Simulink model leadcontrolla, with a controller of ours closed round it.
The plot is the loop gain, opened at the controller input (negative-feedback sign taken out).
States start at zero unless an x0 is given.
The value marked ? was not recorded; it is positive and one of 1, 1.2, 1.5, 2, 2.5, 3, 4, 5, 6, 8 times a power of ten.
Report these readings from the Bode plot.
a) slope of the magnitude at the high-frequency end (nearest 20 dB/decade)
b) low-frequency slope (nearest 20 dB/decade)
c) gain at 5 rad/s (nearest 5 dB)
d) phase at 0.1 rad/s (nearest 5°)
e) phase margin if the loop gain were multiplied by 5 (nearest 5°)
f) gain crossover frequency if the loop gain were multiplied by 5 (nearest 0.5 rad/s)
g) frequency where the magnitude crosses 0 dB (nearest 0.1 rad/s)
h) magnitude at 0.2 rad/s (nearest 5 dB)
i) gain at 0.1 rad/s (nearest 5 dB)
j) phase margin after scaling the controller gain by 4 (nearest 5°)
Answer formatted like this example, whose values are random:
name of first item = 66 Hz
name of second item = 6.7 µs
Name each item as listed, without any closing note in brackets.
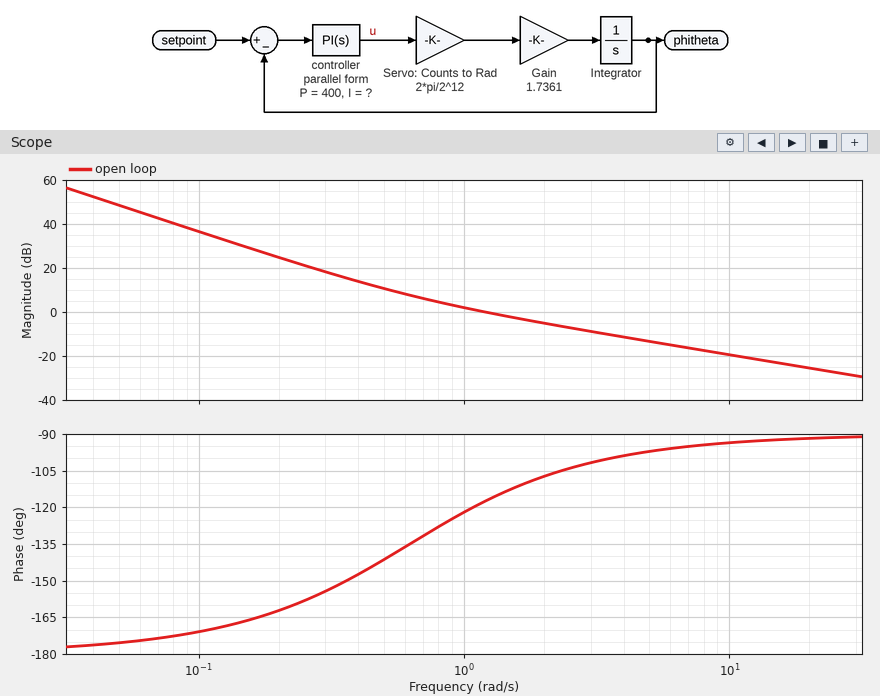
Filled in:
slope of the magnitude at the high-frequency end = -20 dB/decade
low-frequency slope = -40 dB/decade
gain at 5 rad/s = -15 dB
phase at 0.1 rad/s = -170°
phase margin if the loop gain were multiplied by 5 = 85°
gain crossover frequency if the loop gain were multiplied by 5 = 5.5 rad/s
frequency where the magnitude crosses 0 dB = 1.2 rad/s
magnitude at 0.2 rad/s = 25 dB
gain at 0.1 rad/s = 35 dB
phase margin after scaling the controller gain by 4 = 80°
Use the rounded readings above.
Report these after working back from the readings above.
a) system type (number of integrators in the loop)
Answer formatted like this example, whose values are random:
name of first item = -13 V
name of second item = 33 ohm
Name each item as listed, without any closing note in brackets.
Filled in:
system type = 2
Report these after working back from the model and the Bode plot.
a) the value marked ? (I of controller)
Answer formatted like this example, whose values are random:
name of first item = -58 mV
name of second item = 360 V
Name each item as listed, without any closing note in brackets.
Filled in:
the value marked ? = 250
